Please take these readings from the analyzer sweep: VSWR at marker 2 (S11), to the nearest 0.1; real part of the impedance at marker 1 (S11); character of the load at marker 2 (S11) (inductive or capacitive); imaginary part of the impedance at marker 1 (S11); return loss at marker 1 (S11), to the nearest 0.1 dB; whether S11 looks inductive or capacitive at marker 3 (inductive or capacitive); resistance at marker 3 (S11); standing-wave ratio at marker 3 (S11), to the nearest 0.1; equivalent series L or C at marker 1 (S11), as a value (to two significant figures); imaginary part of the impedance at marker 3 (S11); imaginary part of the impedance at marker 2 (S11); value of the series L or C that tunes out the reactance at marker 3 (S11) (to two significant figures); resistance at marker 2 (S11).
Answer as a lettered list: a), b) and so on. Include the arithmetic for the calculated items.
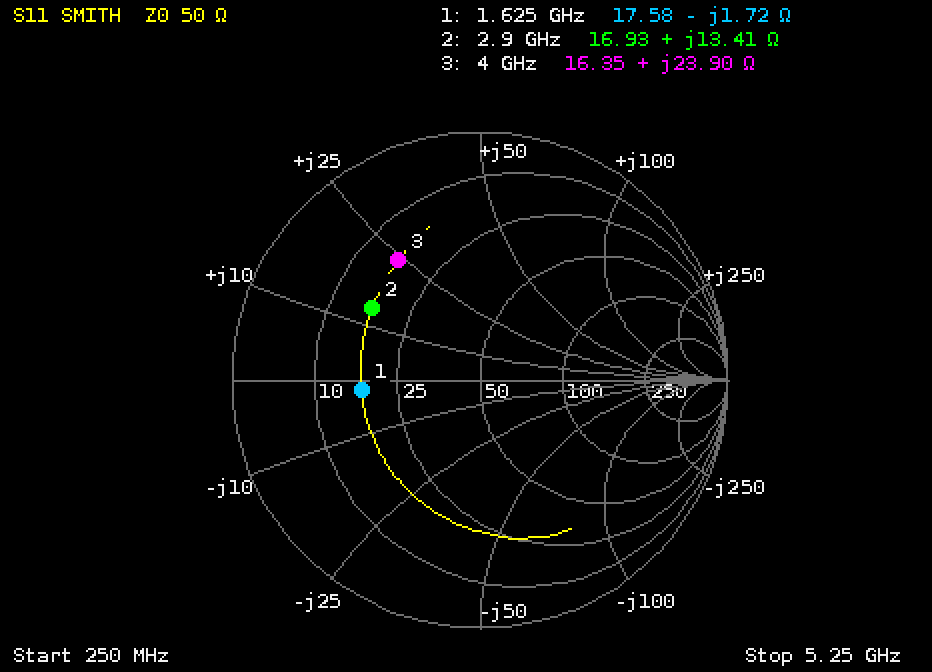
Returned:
a) 3.2
b) 17.58 Ω
c) inductive
d) -1.72 Ω
e) 6.4 dB
f) inductive
g) 16.35 Ω
h) 3.8
i) C = 1/(2π × 1.625 GHz × 1.72 Ω) ≈ 57 pF
j) +23.90 Ω
k) +13.41 Ω
l) C = 1/(2π × 4 GHz × 23.9 Ω) ≈ 1.7 pF
m) 16.93 Ω
